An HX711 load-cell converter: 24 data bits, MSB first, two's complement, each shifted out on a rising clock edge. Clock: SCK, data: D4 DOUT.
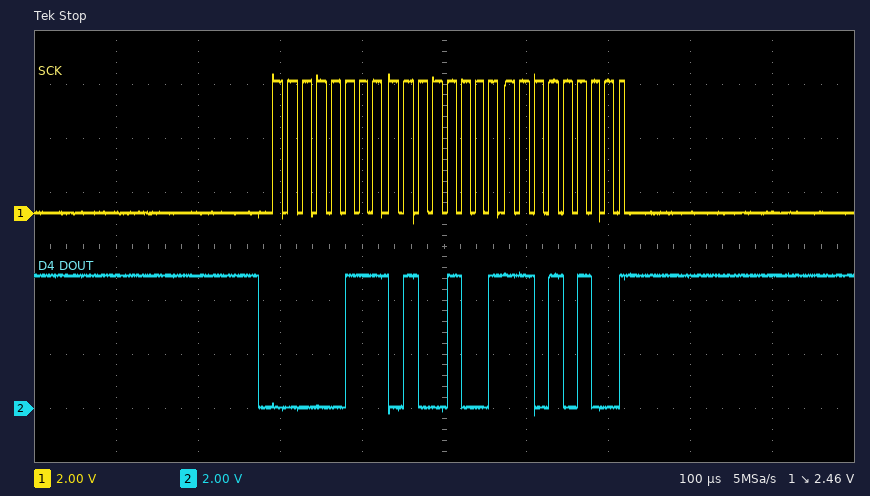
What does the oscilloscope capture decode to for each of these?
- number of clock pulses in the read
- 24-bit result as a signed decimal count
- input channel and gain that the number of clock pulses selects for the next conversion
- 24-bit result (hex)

25
477652
channel A, gain 128
0x0749D4
